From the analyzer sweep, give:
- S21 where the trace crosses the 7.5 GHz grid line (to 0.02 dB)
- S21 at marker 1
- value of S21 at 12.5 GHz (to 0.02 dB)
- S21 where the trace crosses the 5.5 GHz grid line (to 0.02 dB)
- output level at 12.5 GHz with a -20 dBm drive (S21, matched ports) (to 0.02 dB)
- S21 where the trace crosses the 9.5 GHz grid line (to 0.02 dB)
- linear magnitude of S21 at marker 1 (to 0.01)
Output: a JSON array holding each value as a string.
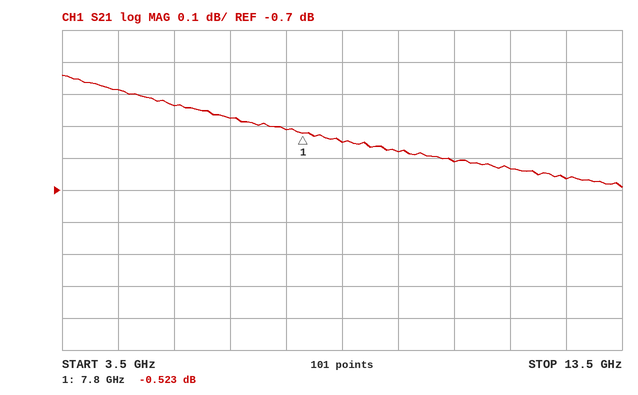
["-0.52 dB", "-0.523 dB", "-0.66 dB", "-0.44 dB", "-20.66 dBm", "-0.58 dB", "0.94"]
